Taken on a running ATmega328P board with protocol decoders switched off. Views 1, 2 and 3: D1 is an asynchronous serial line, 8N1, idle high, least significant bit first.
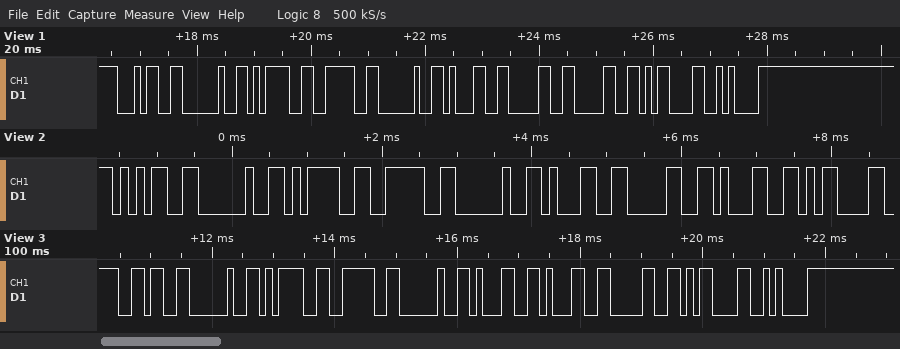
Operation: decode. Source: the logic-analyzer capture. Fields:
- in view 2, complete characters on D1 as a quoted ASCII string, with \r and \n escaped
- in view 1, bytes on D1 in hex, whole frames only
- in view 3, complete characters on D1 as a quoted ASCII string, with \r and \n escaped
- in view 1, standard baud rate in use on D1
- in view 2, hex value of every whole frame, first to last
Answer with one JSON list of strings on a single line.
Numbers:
["\"5 => 101\\r\"", "34 20 3D 3E 20 31 30 30 0D 0A", "\"6 => 110\\r\\n\"", "9600 baud", "0x35 0x20 0x3D 0x3E 0x20 0x31 0x30 0x31 0x0D"]
